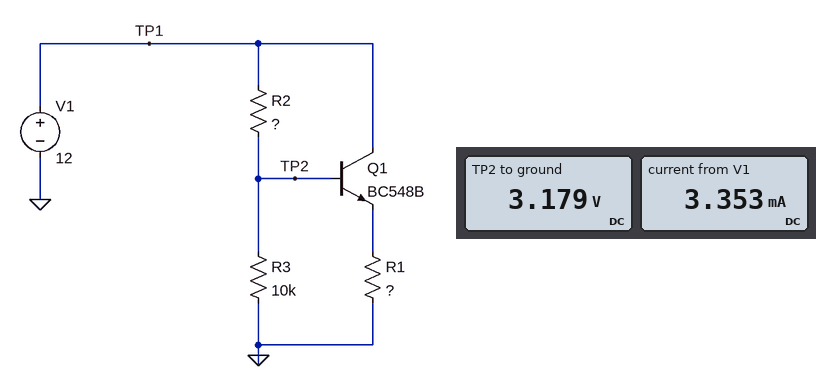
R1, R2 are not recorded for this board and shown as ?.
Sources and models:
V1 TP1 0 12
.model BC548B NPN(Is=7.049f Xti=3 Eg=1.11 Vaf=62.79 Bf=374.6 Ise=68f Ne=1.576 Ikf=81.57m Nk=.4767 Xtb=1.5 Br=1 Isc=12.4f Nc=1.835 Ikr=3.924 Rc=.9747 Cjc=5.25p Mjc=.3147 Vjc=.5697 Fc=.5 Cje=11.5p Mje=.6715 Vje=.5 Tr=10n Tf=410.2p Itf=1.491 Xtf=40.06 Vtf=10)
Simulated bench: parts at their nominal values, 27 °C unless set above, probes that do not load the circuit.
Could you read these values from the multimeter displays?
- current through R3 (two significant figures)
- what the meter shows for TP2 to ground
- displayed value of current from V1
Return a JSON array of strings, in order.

["320 µA", "3.179 V", "3.353 mA"]
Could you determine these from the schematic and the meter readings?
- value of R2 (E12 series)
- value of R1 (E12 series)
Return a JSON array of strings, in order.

["27 kΩ", "820 Ω"]
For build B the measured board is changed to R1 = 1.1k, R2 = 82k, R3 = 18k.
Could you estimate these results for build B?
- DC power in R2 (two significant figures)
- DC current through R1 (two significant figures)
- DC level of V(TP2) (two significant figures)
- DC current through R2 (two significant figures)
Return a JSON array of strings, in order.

["1.2 mW", "1.3 mA", "2.1 V", "120 µA"]
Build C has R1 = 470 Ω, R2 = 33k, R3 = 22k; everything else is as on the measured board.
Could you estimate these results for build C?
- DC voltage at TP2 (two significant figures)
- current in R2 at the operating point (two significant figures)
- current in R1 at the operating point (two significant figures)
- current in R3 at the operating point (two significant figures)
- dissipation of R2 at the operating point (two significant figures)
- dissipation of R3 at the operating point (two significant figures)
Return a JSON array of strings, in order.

["4.5 V", "230 µA", "8.0 mA", "200 µA", "1.7 mW", "920 µW"]
